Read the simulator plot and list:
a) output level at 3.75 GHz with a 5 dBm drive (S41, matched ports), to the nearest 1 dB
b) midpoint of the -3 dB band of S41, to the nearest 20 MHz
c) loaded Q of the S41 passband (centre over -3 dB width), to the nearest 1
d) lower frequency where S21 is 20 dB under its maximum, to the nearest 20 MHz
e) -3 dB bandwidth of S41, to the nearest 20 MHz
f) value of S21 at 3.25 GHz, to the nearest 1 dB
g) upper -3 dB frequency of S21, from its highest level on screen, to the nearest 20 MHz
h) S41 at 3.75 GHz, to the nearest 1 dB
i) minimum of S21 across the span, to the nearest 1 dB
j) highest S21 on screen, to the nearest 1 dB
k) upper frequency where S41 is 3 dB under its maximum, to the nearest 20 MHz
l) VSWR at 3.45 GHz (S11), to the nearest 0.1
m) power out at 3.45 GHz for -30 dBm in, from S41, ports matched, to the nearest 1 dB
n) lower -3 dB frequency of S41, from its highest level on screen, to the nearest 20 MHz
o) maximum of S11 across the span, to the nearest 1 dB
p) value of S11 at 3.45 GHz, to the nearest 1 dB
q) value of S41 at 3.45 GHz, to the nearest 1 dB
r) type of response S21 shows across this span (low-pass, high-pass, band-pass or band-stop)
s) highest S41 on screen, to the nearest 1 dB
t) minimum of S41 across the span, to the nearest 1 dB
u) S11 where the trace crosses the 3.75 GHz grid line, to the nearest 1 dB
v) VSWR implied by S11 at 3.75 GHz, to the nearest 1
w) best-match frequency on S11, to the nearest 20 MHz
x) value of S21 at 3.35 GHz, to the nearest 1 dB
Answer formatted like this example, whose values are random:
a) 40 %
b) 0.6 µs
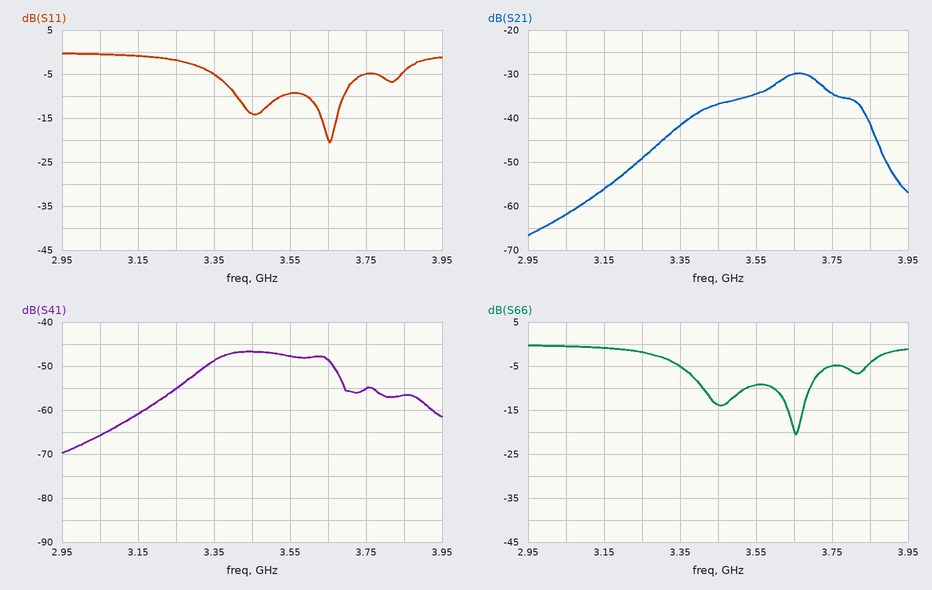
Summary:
a) -50 dBm
b) 3.50 GHz
c) 11
d) 3.24 GHz
e) 320 MHz
f) -49 dB
g) 3.72 GHz
h) -55 dB
i) -67 dB
j) -30 dB
k) 3.66 GHz
l) 1.5
m) -77 dBm
n) 3.34 GHz
o) 0 dB
p) -14 dB
q) -47 dB
r) band-pass
s) -47 dB
t) -70 dB
u) -5 dB
v) 4
w) 3.66 GHz
x) -42 dB
